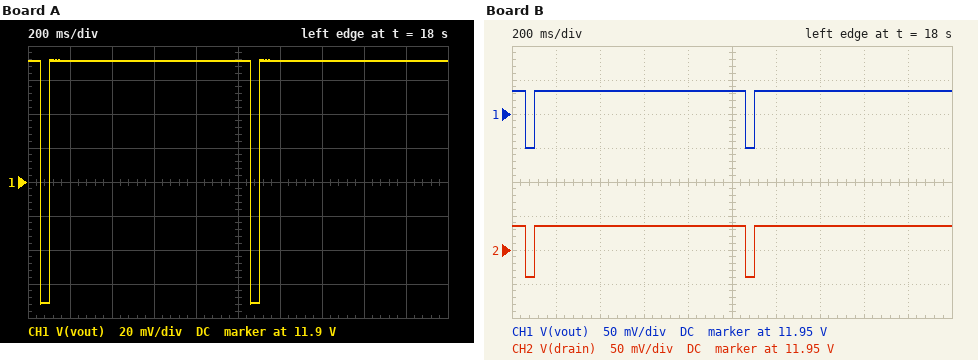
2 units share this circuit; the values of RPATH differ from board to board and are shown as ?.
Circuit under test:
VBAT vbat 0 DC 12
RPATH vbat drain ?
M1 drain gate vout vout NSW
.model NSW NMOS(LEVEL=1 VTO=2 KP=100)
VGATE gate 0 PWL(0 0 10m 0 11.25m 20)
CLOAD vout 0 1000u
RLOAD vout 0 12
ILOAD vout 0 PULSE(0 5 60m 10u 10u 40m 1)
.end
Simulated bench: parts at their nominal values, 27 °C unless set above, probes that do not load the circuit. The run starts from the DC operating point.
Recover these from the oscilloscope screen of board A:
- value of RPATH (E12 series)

0.027 Ω
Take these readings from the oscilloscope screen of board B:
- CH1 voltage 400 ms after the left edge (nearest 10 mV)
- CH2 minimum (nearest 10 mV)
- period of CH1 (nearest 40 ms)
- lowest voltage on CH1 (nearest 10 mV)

11.98 V
11.91 V
1.00 s
11.90 V
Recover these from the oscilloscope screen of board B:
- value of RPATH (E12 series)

0.015 Ω
